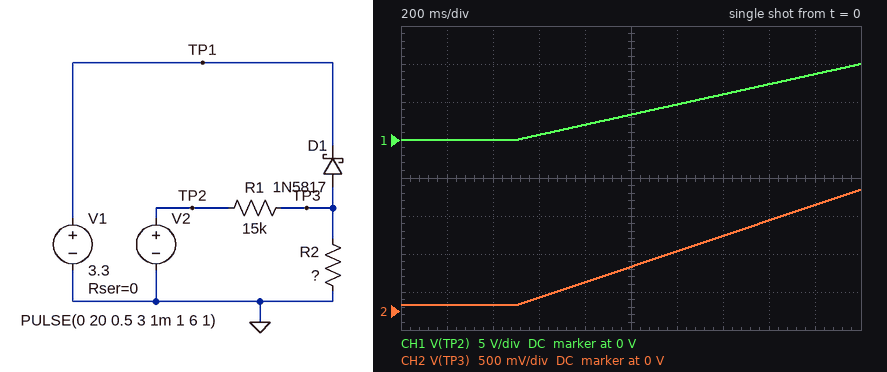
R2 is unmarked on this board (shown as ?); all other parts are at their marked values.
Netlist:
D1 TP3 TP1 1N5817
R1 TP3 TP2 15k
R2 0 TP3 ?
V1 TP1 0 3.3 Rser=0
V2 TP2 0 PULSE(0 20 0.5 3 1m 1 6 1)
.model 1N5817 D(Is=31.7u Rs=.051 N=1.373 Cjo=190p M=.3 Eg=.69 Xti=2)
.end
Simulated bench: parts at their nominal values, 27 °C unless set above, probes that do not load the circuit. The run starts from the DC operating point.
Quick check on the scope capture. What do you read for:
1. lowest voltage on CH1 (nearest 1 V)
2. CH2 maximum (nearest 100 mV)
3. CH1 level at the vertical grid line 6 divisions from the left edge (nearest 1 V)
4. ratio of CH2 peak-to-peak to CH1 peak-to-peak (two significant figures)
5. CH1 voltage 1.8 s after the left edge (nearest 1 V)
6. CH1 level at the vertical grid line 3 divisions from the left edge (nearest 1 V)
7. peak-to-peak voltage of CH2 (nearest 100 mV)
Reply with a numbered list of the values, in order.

1. 0 V
2. 1.6 V
3. 5 V
4. 0.15
5. 9 V
6. 1 V
7. 1.5 V
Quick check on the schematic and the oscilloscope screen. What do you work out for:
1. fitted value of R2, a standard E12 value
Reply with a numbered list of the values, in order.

1. 2.7 kΩ
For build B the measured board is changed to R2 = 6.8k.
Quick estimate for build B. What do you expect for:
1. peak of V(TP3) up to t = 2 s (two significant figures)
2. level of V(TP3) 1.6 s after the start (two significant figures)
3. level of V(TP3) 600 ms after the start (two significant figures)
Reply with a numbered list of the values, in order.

1. 3.2 V
2. 2.4 V
3. 360 mV
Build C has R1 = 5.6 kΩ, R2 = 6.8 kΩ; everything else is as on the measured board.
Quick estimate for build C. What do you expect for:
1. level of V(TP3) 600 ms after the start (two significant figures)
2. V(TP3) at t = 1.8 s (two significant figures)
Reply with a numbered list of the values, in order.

1. 460 mV
2. 3.4 V
